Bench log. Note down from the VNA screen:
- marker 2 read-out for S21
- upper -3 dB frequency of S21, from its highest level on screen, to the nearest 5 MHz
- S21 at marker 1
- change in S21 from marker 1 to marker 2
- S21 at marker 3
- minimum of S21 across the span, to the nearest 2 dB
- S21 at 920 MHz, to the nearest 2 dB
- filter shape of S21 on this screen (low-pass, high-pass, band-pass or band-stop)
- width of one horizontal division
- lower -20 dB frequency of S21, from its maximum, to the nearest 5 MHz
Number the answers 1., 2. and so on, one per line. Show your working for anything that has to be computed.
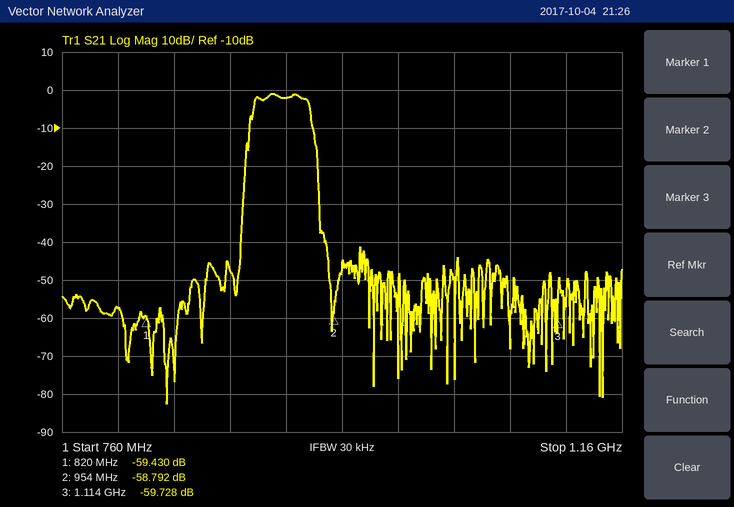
1. -58.792 dB
2. 935 MHz
3. -59.430 dB
4. -58.792 − (-59.43) = 0.638 dB
5. -59.728 dB
6. -82 dB
7. -2 dB
8. band-pass
9. 40 MHz
10. 890 MHz
